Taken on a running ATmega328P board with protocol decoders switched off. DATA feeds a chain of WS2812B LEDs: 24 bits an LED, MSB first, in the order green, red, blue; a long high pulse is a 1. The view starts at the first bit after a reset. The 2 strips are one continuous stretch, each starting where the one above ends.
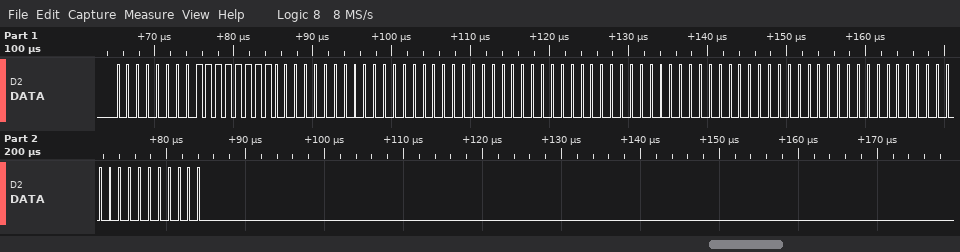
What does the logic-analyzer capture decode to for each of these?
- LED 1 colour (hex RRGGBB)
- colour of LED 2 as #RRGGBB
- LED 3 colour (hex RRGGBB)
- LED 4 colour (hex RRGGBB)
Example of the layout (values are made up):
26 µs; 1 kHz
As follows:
#FF0000; #000000; #000000; #000000
